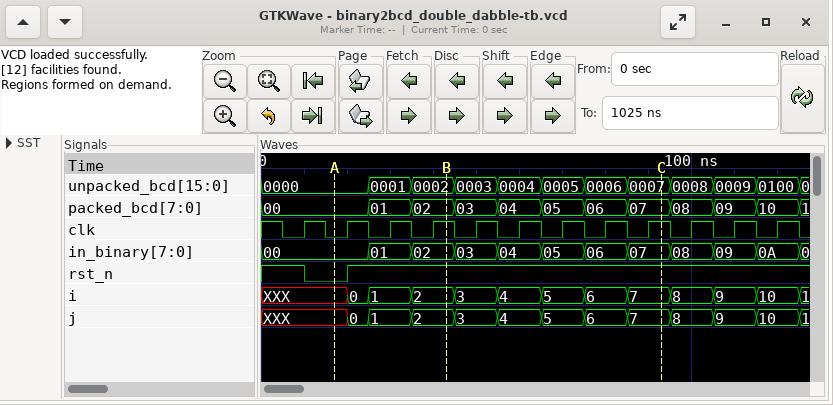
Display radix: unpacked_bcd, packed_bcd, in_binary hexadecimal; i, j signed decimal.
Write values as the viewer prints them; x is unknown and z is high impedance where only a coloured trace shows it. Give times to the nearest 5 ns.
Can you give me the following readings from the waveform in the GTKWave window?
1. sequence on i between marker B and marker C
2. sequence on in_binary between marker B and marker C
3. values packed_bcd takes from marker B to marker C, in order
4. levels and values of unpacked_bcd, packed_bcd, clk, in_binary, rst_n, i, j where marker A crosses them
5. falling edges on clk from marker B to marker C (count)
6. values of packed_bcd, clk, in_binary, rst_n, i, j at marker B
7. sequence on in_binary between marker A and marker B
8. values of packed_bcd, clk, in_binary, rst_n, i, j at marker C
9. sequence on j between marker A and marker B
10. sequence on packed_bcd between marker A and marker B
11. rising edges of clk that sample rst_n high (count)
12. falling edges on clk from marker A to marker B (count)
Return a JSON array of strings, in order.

["2, 3, 4, 5, 6, 7", "02, 03, 04, 05, 06, 07", "02, 03, 04, 05, 06, 07", "unpacked_bcd=0000, packed_bcd=00, clk=0, in_binary=00, rst_n=0, i=XXX, j=XXX", "5", "packed_bcd=02, clk=1, in_binary=02, rst_n=1, i=2, j=2", "00, 01, 02", "packed_bcd=07, clk=1, in_binary=07, rst_n=1, i=7, j=7", "XXX, 0, 1, 2", "00, 01, 02", "11", "2"]
